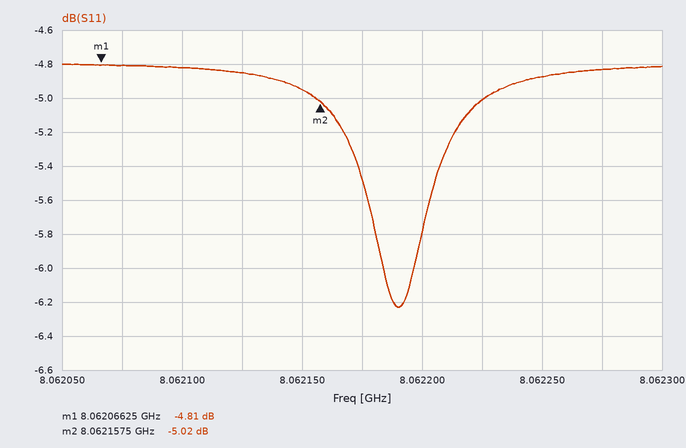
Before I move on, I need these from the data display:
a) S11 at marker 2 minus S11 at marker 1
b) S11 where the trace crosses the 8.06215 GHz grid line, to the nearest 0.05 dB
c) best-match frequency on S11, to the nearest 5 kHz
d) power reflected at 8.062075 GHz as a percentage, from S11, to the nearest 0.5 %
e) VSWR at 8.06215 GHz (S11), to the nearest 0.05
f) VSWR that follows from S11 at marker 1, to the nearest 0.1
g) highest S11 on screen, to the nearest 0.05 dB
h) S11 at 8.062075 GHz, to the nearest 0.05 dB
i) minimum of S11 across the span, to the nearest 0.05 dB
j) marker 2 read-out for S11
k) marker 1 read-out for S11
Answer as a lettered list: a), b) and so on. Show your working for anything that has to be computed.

a) -5.02 − (-4.81) = -0.21 dB
b) -4.95 dB
c) 8.062190 GHz
d) 10^(-4.8/10) ≈ 33.1 %, so 33.0 % to the nearest 0.5 %
e) |Γ| = 10^(-4.95/20) = 0.5656; VSWR = (1 + 0.5656)/(1 − 0.5656) ≈ 3.60
f) (1 + 0.5748)/(1 − 0.5748) ≈ 3.7
g) -4.80 dB
h) -4.80 dB
i) -6.25 dB
j) -5.02 dB
k) -4.81 dB
